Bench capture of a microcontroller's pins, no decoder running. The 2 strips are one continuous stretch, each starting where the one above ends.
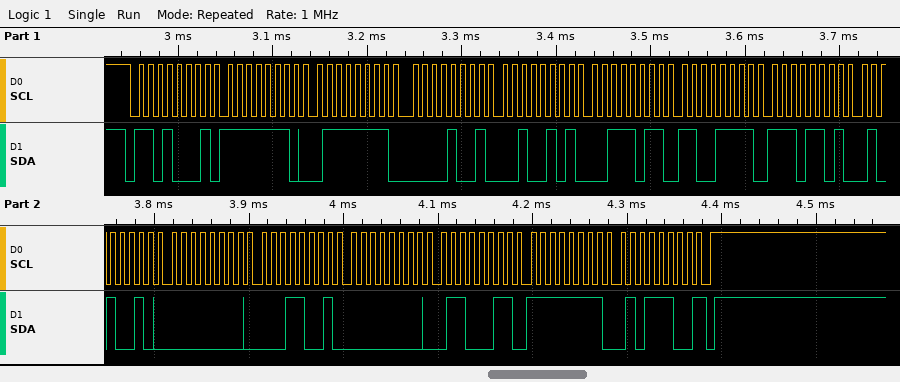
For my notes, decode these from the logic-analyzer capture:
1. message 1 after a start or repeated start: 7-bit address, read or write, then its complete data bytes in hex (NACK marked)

0x68 read: FE 7F 09 25 3B CF ED 52 00 19 00 63 FF 5C NACK
